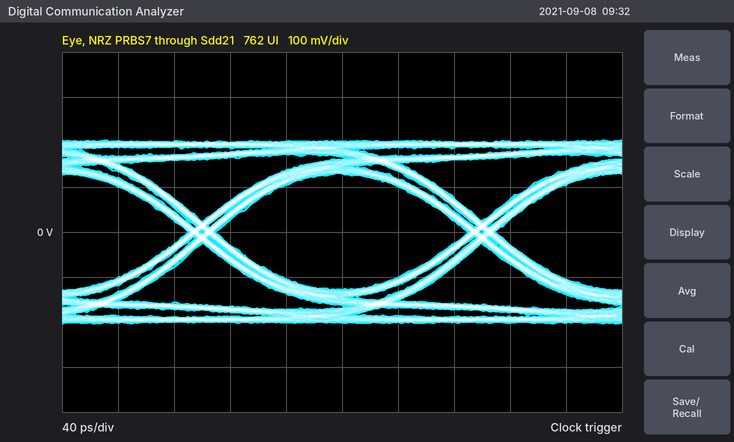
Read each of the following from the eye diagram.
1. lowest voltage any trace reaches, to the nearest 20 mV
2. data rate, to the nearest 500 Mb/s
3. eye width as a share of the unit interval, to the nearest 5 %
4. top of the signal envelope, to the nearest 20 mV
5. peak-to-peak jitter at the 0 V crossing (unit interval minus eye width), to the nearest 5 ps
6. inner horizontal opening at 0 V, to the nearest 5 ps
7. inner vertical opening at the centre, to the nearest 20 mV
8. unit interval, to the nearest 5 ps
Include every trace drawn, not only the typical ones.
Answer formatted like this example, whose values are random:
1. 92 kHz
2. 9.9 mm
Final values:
1. -200 mV
2. 5.0 Gb/s
3. 90 %
4. 200 mV
5. 20 ps
6. 180 ps
7. 260 mV
8. 200 ps
